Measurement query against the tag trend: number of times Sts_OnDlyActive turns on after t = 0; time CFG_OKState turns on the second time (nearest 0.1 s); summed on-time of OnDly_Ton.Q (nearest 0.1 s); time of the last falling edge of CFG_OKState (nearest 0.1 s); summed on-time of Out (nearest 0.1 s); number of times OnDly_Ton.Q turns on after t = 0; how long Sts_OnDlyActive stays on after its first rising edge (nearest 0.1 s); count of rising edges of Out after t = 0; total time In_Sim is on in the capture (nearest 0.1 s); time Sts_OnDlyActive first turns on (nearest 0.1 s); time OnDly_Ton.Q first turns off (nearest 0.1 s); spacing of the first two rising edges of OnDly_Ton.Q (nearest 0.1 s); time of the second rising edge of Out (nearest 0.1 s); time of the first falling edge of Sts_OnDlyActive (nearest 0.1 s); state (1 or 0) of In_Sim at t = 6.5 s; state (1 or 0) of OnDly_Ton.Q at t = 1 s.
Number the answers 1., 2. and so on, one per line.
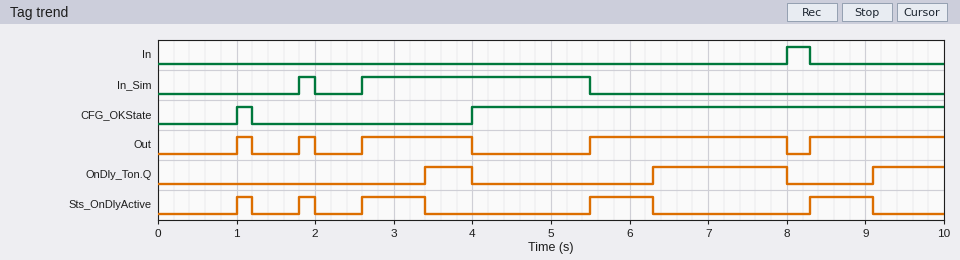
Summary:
1. 5
2. 4.0 s
3. 3.2 s
4. 1.2 s
5. 6.0 s
6. 3
7. 0.2 s
8. 5
9. 3.1 s
10. 1.0 s
11. 4.0 s
12. 2.9 s
13. 1.8 s
14. 1.2 s
15. 0
16. 0
